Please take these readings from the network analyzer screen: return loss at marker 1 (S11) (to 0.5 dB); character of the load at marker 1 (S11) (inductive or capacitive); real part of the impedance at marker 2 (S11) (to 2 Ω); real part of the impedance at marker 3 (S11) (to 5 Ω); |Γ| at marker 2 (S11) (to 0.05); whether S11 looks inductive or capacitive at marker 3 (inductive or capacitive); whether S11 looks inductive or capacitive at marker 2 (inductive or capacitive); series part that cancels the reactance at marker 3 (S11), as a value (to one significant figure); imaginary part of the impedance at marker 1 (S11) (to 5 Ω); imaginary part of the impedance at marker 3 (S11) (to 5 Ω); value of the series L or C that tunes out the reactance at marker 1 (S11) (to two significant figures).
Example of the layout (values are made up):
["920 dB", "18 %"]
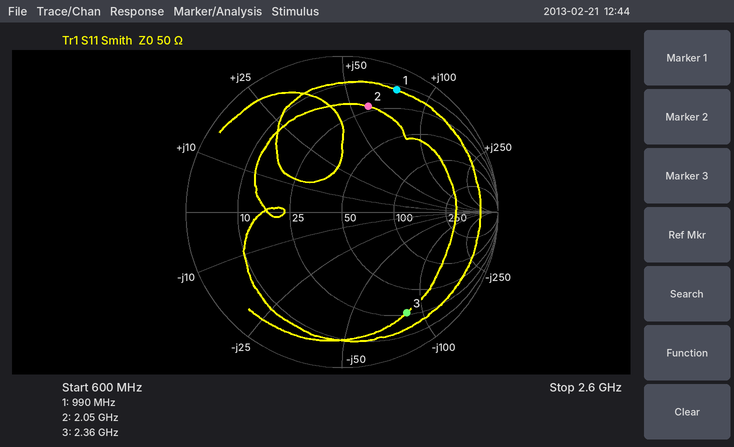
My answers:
["1.5 dB", "inductive", "22 Ω", "25 Ω", "0.70", "capacitive", "inductive", "6 nH", "+75 Ω", "-85 Ω", "2.1 pF"]
